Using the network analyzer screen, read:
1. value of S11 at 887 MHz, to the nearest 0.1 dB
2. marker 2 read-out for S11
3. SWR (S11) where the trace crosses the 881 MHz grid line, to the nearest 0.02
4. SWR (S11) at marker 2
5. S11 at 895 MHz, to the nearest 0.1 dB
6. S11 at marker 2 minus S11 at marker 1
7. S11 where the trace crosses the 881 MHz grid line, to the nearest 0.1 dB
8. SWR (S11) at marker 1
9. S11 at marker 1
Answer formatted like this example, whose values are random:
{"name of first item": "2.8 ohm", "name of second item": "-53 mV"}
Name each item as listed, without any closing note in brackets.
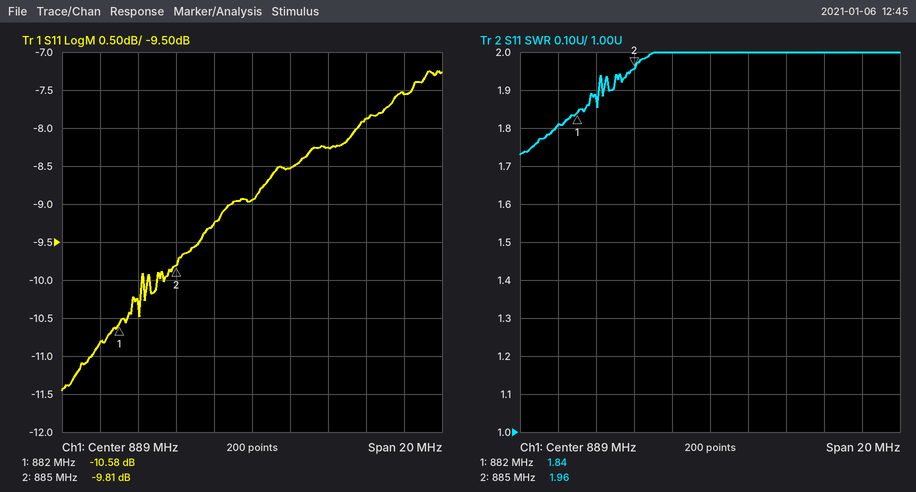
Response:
{"value of S11 at 887 MHz, to the nearest 0.1 dB": "-9.3 dB", "marker 2 read-out for S11": "-9.81 dB", "SWR (S11) where the trace crosses the 881 MHz grid line, to the nearest 0.02": "1.80", "SWR (S11) at marker 2": "1.96", "S11 at 895 MHz, to the nearest 0.1 dB": "-7.9 dB", "S11 at marker 2 minus S11 at marker 1": "0.77 dB", "S11 where the trace crosses the 881 MHz grid line, to the nearest 0.1 dB": "-10.8 dB", "SWR (S11) at marker 1": "1.84", "S11 at marker 1": "-10.58 dB"}
